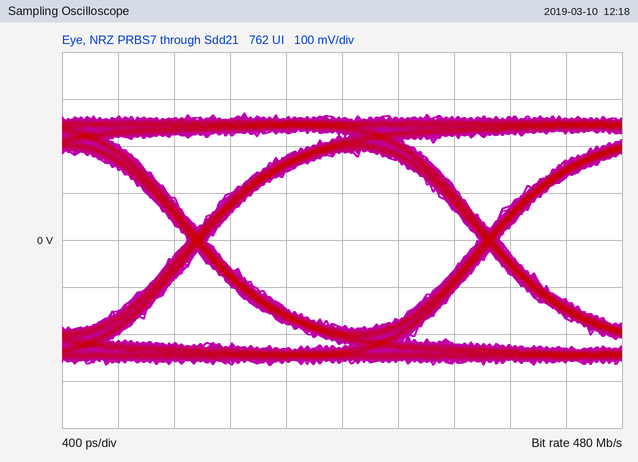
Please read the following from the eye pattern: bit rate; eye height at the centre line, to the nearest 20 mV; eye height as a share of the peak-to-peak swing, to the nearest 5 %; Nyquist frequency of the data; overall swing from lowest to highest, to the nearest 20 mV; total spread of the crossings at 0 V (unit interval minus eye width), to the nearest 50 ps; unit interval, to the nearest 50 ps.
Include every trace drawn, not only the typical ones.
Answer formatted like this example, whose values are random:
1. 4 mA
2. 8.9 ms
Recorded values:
1. 480 Mb/s
2. 380 mV
3. 70 %
4. 240 MHz
5. 540 mV
6. 150 ps
7. 2.10 ns
